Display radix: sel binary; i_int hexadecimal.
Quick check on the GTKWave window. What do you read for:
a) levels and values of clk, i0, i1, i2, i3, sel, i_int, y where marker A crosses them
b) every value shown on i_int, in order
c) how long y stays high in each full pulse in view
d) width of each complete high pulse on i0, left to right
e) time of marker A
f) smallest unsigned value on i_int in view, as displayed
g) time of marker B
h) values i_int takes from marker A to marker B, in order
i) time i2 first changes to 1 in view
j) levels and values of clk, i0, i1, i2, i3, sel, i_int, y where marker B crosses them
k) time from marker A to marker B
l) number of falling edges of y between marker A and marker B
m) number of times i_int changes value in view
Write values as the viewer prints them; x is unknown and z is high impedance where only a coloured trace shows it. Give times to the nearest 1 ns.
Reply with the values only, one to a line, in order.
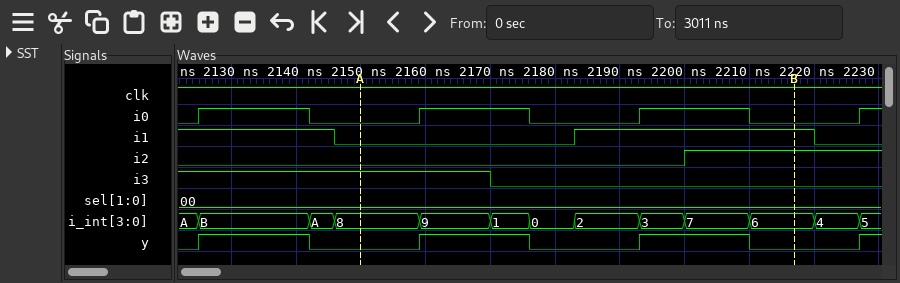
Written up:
clk=1, i0=0, i1=0, i2=0, i3=1, sel=00, i_int=8, y=0
A, B, A, 8, 9, 1, 0, 2, 3, 7, 6, 4, 5
17 ns, 17 ns, 17 ns
17 ns, 17 ns, 17 ns
2150 ns
0
2217 ns
8, 9, 1, 0, 2, 3, 7, 6
2200 ns
clk=1, i0=0, i1=1, i2=1, i3=0, sel=00, i_int=6, y=0
67 ns
2
12
